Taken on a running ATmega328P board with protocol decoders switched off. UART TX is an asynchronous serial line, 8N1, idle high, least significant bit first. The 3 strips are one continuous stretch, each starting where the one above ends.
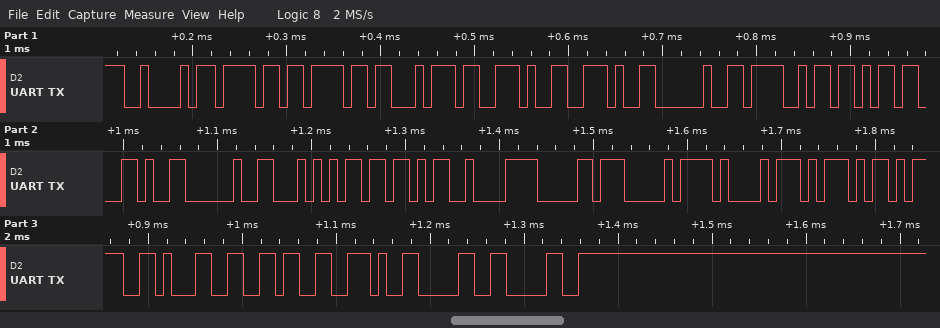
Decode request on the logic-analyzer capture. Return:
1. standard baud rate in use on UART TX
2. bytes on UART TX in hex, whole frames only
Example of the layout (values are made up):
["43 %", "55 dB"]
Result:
["115200 baud", "42 6F 6F 74 2E 2E 20 4F 6B 2C 20 54 5B C2 B0 D0 A1 5D 3D 31 36 2E 30 30"]
